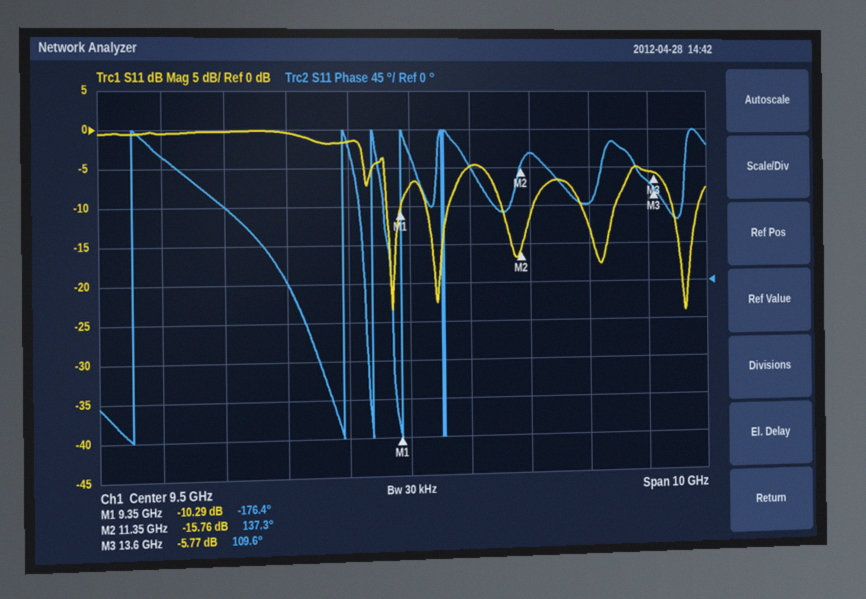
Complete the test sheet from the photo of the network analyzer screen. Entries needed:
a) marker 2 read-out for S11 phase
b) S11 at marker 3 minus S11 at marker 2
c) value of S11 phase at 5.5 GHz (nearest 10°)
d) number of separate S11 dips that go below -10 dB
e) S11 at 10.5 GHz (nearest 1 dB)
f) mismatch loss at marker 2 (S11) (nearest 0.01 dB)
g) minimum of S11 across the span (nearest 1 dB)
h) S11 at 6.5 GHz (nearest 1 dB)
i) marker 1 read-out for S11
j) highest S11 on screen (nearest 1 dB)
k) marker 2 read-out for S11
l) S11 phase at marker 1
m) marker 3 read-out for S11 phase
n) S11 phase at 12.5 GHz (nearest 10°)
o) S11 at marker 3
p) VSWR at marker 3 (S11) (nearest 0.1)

137.3°
9.99 dB
150°
5
-5 dB
0.12 dB
-24 dB
0 dB
-10.29 dB
0 dB
-15.76 dB
-176.4°
109.6°
90°
-5.77 dB
3.1
